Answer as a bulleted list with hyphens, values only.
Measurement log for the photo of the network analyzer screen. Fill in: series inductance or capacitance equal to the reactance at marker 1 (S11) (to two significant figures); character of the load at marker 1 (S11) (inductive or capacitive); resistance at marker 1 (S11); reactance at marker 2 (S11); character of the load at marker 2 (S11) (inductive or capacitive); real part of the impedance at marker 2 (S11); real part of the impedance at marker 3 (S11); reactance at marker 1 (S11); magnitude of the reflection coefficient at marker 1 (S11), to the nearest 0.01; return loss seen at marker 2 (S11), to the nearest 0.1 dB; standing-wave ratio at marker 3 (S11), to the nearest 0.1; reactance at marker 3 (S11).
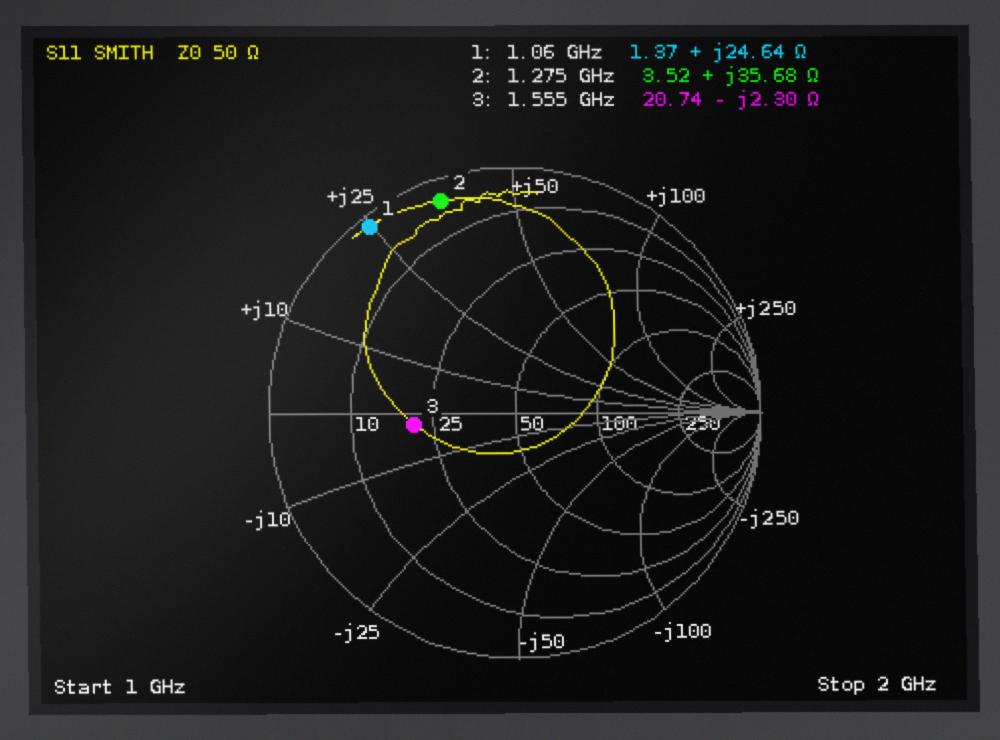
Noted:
- 3.7 nH
- inductive
- 1.37 Ω
- +35.68 Ω
- inductive
- 3.52 Ω
- 20.74 Ω
- +24.64 Ω
- 0.96
- 0.8 dB
- 2.4
- -2.30 Ω
